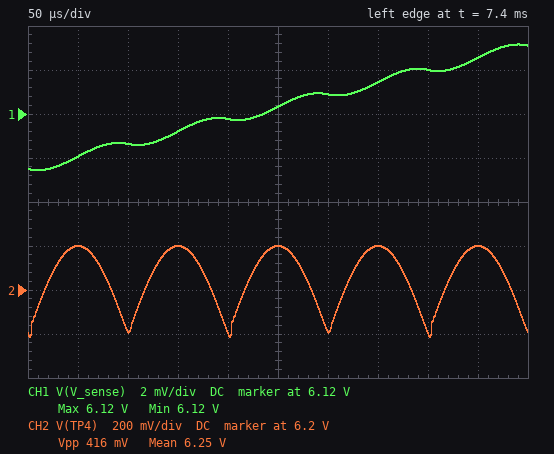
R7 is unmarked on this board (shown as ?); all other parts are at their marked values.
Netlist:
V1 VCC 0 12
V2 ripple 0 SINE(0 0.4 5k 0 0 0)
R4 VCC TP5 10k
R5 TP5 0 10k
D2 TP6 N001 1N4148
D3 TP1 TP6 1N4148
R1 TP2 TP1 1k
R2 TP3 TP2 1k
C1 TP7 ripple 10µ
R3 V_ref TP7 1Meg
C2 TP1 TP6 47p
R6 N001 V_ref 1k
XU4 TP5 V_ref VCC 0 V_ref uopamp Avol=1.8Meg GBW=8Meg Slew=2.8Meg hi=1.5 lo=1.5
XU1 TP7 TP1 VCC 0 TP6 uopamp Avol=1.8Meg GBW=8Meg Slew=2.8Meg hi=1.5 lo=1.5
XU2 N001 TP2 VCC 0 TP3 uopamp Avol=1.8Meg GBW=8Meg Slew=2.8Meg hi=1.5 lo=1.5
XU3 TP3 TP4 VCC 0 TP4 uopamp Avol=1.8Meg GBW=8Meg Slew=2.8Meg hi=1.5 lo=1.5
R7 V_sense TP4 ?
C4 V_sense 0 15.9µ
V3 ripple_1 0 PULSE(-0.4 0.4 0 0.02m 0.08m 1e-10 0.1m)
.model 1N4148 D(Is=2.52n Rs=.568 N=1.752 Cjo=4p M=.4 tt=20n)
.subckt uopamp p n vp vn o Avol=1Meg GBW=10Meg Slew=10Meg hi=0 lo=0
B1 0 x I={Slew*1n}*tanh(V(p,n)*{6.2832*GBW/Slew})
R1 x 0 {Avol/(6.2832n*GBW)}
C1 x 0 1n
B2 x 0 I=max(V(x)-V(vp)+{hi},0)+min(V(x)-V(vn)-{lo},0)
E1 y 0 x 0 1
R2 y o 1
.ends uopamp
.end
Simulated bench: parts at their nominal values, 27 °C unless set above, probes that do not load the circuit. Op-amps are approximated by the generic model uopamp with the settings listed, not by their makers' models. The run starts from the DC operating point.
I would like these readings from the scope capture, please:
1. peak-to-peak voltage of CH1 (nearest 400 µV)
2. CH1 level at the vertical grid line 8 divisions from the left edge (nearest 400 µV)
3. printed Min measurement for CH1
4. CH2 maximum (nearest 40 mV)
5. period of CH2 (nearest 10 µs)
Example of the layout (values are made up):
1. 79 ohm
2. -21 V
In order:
1. 5.6 mV
2. 6.1220 V
3. 6.12 V
4. 6.40 V
5. 100 µs
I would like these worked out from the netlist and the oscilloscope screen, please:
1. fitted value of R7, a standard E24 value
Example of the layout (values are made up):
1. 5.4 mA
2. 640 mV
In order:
1. 750 Ω
